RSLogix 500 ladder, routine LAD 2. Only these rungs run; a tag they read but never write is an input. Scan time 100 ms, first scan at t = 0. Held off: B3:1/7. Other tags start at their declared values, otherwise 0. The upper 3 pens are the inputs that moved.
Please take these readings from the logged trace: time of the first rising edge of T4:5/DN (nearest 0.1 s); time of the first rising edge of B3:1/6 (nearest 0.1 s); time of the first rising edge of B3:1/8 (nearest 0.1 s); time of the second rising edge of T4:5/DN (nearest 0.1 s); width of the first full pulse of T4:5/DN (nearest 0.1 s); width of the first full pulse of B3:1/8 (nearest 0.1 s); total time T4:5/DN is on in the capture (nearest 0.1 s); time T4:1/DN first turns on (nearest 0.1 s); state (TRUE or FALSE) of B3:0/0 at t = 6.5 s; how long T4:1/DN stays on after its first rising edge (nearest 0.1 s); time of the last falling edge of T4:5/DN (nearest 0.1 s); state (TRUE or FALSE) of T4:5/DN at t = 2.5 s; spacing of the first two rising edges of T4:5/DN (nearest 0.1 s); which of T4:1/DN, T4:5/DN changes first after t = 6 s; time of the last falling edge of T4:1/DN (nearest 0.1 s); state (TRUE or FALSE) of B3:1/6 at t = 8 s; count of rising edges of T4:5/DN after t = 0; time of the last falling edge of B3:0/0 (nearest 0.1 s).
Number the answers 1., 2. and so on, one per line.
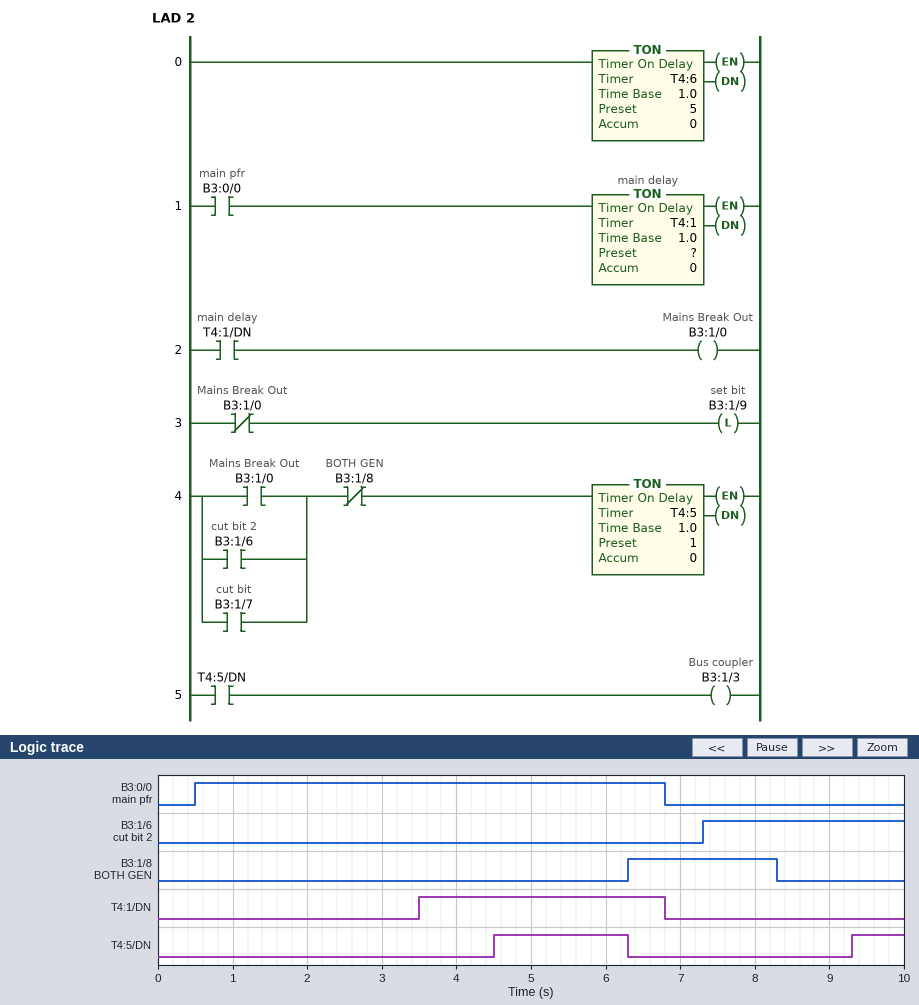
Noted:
1. 4.5 s
2. 7.3 s
3. 6.3 s
4. 9.3 s
5. 1.8 s
6. 2.0 s
7. 2.5 s
8. 3.5 s
9. TRUE
10. 3.3 s
11. 6.3 s
12. FALSE
13. 4.8 s
14. T4:5/DN
15. 6.8 s
16. TRUE
17. 2
18. 6.8 s
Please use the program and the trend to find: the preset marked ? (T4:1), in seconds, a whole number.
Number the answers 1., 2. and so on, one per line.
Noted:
1. 3 s
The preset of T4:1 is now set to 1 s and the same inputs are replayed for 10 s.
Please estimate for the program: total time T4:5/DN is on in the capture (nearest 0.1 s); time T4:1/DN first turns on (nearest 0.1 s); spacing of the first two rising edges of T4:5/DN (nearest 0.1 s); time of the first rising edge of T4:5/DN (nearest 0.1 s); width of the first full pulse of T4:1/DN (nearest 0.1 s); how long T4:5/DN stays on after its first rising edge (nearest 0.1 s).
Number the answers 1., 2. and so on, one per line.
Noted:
1. 4.5 s
2. 1.5 s
3. 6.8 s
4. 2.5 s
5. 5.3 s
6. 3.8 s
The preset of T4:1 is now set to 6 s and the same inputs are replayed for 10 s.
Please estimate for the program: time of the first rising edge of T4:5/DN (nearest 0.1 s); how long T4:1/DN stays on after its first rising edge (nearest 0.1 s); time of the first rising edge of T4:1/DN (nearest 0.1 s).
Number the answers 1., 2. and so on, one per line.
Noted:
1. 9.3 s
2. 0.3 s
3. 6.5 s
